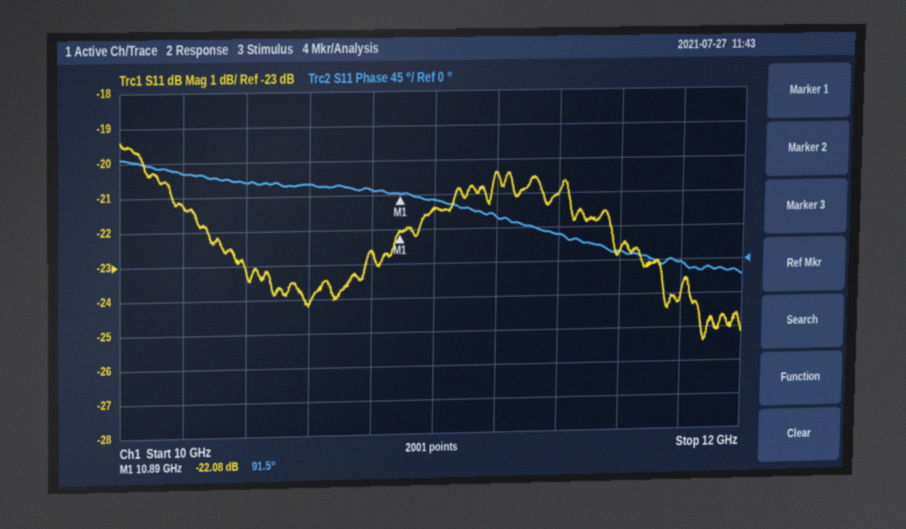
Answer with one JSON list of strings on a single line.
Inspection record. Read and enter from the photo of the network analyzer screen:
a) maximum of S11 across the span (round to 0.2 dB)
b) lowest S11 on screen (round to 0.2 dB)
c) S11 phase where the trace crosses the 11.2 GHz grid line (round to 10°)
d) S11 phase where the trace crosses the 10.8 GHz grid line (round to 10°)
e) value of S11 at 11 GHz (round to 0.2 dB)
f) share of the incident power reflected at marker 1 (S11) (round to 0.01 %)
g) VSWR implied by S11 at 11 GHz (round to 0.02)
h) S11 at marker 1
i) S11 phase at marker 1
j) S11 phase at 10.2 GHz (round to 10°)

["-19.4 dB", "-25.4 dB", "60°", "100°", "-21.4 dB", "0.62 %", "1.18", "-22.08 dB", "91.5°", "120°"]
